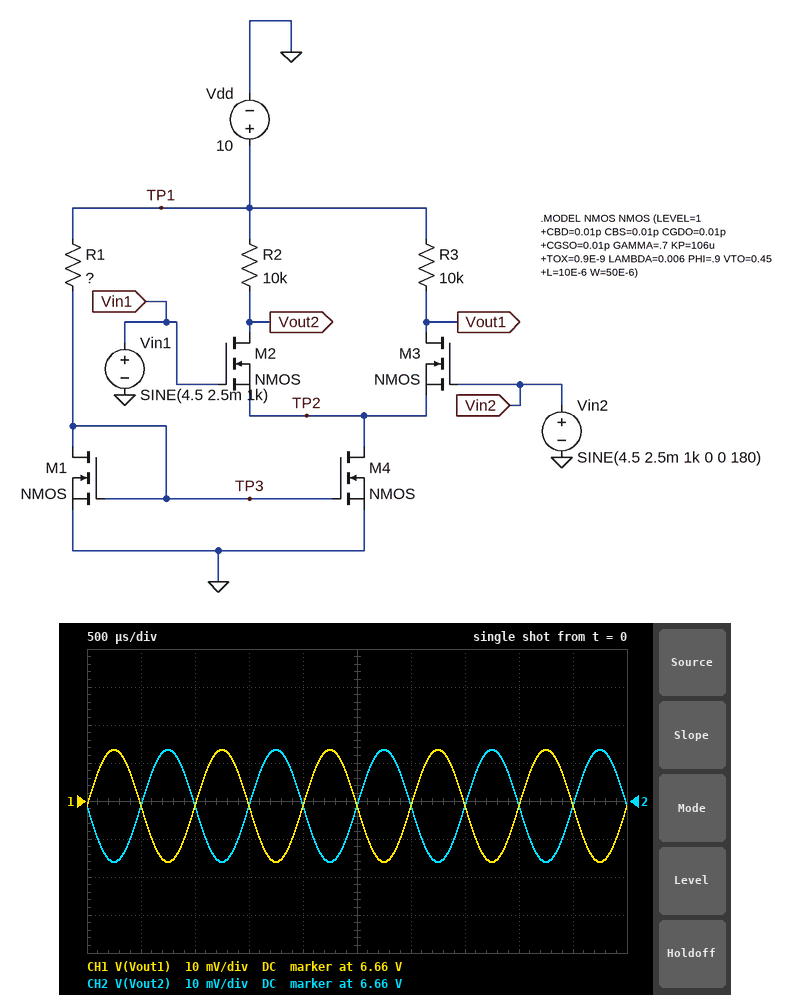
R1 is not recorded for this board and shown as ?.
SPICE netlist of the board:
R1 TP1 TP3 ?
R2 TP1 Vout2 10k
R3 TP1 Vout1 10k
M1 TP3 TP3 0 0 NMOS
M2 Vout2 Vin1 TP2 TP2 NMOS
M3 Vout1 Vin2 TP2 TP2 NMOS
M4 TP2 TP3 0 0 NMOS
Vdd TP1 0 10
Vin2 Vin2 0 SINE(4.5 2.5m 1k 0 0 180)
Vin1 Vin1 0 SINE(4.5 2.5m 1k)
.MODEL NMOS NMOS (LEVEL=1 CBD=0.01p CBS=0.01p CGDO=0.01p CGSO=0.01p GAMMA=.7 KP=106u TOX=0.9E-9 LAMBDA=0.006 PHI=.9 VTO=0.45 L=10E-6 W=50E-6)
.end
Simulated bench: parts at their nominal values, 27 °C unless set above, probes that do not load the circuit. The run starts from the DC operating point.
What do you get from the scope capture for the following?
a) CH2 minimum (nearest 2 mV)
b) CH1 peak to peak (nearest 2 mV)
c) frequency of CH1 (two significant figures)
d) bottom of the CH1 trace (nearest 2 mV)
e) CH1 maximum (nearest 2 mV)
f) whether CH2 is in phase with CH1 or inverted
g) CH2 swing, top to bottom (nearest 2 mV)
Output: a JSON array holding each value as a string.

["6.644 V", "30 mV", "1.0 kHz", "6.644 V", "6.674 V", "inverted", "30 mV"]
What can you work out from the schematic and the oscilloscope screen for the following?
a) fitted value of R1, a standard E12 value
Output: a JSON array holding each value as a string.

["12 kΩ"]
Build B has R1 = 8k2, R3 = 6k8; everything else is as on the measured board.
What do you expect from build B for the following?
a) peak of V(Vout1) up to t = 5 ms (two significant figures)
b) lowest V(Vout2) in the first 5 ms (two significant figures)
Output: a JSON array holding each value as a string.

["6.8 V", "5.3 V"]
